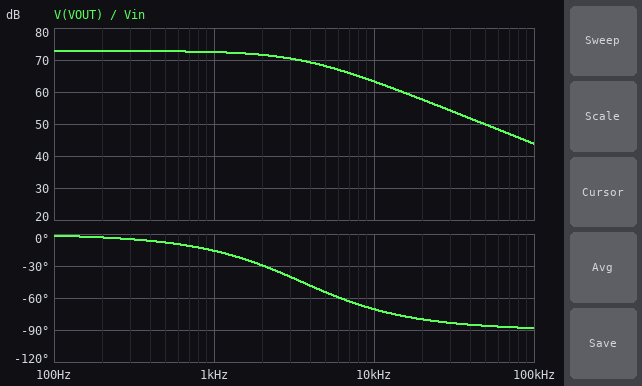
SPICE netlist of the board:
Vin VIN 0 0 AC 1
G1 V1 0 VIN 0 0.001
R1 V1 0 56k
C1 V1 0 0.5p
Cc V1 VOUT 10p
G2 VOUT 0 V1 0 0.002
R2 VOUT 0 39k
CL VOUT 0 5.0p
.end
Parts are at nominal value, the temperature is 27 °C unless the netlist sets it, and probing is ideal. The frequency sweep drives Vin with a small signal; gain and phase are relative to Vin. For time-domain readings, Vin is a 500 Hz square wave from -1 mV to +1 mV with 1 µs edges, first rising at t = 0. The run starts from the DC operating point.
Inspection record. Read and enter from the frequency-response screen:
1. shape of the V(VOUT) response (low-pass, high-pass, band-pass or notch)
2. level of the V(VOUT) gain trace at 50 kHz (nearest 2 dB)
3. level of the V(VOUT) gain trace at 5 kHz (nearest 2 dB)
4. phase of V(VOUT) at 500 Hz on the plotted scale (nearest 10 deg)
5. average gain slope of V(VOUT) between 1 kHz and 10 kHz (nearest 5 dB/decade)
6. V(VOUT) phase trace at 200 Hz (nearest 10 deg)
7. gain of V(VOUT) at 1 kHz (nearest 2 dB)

low-pass
50 dB
68 dB
-10 deg
-10 dB/decade
0 deg
72 dB
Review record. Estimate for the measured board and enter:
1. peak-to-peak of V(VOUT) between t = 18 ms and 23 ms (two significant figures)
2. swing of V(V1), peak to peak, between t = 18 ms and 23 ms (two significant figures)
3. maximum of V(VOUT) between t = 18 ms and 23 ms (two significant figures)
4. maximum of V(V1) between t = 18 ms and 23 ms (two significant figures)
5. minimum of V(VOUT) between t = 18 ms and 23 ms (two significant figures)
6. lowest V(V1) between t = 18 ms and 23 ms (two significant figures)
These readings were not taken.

8.7 V
110 mV
4.4 V
56 mV
-4.4 V
-56 mV
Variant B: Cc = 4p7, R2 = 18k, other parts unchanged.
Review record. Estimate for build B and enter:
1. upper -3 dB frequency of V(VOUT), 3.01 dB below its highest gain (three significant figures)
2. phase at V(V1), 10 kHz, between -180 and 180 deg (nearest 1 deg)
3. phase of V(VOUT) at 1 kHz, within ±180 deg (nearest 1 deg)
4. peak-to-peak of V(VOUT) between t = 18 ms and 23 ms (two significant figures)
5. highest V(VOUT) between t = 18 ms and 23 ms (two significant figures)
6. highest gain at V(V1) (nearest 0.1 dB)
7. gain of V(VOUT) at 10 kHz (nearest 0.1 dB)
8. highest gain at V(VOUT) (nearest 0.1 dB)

16.0 kHz
149 deg
-4 deg
4.0 V
2.0 V
35.0 dB
64.7 dB
66.1 dB
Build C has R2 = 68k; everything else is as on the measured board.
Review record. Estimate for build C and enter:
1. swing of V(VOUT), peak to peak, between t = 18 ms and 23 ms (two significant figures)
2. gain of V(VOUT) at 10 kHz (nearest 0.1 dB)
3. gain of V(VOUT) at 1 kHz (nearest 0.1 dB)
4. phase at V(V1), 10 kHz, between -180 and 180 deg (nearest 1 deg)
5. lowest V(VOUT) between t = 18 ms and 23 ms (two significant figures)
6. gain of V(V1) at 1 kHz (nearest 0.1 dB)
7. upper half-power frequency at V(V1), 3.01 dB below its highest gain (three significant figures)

15 V
63.7 dB
76.7 dB
105 deg
-7.6 V
34.0 dB
2.05 kHz
